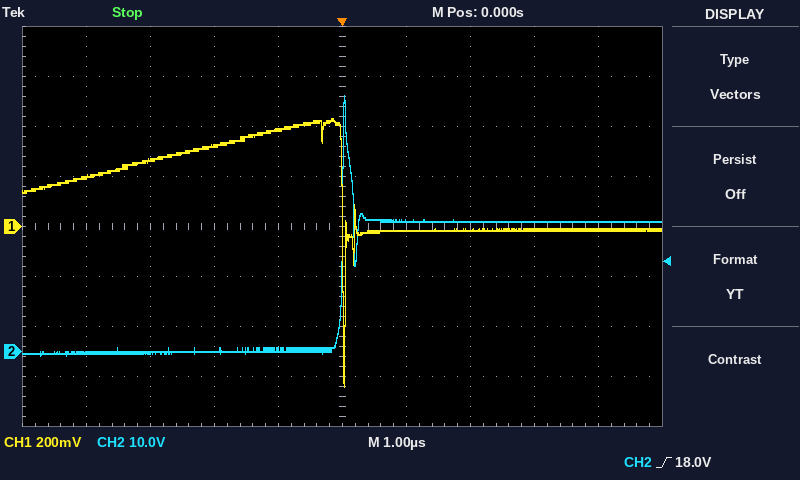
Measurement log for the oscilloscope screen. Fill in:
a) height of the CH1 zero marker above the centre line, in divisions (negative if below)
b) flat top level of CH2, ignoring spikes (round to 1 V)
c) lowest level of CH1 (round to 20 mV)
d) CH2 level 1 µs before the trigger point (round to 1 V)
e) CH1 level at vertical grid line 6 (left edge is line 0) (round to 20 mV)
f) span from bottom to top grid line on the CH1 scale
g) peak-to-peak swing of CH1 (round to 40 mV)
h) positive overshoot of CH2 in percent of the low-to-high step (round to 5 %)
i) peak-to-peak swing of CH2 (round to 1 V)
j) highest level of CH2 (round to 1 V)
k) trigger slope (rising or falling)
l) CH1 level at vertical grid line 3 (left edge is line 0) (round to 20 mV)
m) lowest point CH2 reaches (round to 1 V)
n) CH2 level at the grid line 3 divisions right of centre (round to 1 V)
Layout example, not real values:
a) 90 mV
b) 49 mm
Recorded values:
a) 0.0 div
b) 26 V
c) -640 mV
d) 0 V
e) -20 mV
f) 1.6 V
g) 1.08 V
h) 95 %
i) 52 V
j) 51 V
k) rising
l) 320 mV
m) -1 V
n) 26 V
